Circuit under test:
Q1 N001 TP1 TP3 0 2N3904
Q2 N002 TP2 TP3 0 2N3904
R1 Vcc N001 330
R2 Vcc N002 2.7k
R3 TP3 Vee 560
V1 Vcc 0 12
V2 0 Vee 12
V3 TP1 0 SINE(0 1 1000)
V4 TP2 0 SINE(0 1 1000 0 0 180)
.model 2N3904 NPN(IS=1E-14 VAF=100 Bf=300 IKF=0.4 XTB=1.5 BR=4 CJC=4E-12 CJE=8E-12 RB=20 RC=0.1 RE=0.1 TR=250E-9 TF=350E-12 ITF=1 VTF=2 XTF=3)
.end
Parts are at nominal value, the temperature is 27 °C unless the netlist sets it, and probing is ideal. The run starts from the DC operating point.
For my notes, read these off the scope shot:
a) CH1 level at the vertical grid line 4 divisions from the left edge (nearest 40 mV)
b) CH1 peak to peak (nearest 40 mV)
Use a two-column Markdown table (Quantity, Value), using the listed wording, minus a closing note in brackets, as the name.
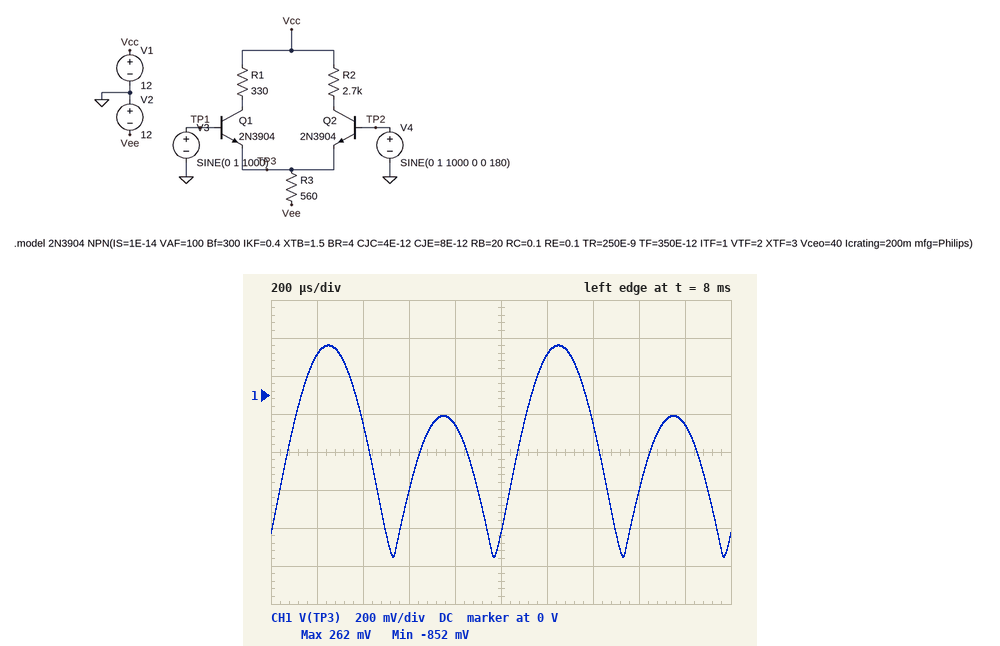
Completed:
| Quantity | Value |
|---|---|
| CH1 level at the vertical grid line 4 divisions from the left edge | -160 mV |
| CH1 peak to peak | 1.12 V |
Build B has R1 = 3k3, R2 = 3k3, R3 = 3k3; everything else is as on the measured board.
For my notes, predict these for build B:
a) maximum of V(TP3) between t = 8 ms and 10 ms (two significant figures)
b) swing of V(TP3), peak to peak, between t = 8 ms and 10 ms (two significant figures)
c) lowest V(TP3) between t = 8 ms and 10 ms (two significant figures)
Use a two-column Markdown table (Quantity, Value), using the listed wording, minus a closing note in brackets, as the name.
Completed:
| Quantity | Value |
|---|---|
| maximum of V(TP3) between t = 8 ms and 10 ms | 300 mV |
| swing of V(TP3), peak to peak, between t = 8 ms and 10 ms | 970 mV |
| lowest V(TP3) between t = 8 ms and 10 ms | -670 mV |
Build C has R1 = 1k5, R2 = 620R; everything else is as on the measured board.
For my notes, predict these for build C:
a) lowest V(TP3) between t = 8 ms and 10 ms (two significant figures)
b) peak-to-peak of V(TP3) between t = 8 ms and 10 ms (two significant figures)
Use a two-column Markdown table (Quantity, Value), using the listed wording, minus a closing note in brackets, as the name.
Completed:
| Quantity | Value |
|---|---|
| lowest V(TP3) between t = 8 ms and 10 ms | -810 mV |
| peak-to-peak of V(TP3) between t = 8 ms and 10 ms | 1.0 V |
